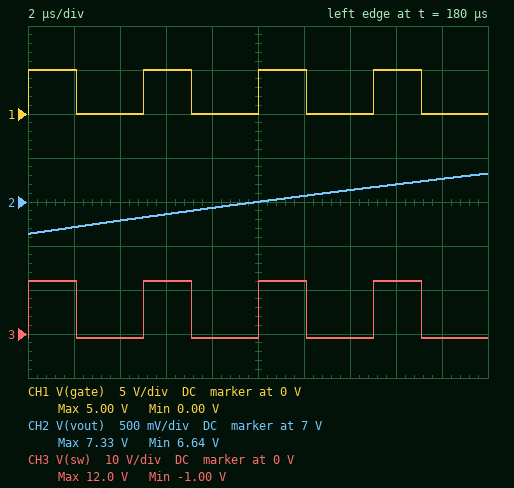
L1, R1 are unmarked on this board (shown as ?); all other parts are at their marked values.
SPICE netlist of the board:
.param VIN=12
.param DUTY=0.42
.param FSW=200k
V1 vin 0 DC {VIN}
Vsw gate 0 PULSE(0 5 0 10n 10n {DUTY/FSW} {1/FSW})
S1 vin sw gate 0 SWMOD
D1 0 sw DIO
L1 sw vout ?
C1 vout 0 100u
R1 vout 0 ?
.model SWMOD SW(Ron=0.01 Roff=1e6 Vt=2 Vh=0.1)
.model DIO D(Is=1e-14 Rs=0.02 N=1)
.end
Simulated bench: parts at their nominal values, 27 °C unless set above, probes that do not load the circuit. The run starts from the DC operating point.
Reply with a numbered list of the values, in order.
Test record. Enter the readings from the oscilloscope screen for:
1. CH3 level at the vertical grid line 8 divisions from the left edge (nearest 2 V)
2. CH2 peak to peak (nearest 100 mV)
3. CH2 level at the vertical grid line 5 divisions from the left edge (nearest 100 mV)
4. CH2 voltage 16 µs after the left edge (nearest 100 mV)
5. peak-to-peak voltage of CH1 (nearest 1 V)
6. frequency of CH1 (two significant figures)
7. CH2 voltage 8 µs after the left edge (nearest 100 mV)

1. 12 V
2. 700 mV
3. 7.0 V
4. 7.2 V
5. 5 V
6. 200 kHz
7. 6.9 V
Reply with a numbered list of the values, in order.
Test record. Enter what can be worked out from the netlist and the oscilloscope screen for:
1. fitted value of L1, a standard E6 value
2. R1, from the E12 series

1. 68 µH
2. 6.8 Ω
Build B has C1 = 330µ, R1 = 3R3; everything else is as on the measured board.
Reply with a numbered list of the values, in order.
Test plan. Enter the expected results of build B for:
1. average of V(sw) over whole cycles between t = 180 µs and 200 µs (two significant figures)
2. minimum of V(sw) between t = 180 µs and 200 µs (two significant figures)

1. 4.4 V
2. -1.1 V
